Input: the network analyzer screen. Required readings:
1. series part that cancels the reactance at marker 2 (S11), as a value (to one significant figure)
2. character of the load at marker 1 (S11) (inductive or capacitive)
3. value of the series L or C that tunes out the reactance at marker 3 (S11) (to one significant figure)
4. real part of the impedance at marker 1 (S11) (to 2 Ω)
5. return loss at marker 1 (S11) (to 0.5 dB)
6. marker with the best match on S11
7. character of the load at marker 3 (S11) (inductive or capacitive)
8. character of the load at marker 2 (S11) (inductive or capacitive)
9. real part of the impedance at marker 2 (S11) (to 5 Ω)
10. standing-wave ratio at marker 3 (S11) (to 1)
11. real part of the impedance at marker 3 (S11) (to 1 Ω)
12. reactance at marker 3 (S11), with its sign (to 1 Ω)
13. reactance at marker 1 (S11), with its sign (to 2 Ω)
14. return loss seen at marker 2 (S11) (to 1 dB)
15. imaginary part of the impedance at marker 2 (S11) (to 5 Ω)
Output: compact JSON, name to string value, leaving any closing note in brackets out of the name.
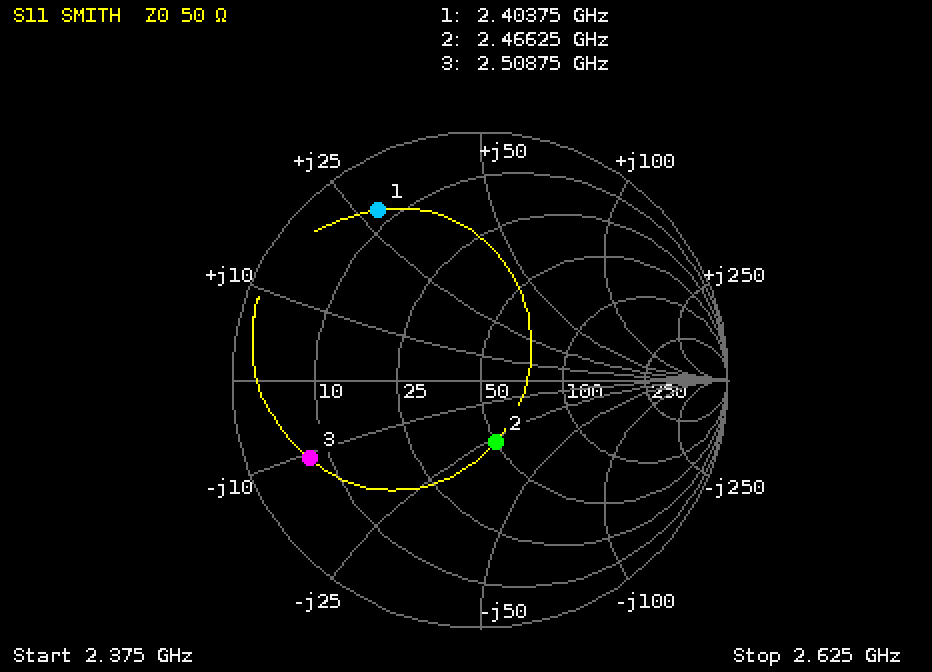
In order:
{"series part that cancels the reactance at marker 2 (S11), as a value": "2 nH", "character of the load at marker 1 (S11)": "inductive", "value of the series L or C that tunes out the reactance at marker 3 (S11)": "700 pH", "real part of the impedance at marker 1 (S11)": "8 Ω", "return loss at marker 1 (S11)": "2.0 dB", "marker with the best match on S11": "marker 2", "character of the load at marker 3 (S11)": "capacitive", "character of the load at marker 2 (S11)": "capacitive", "real part of the impedance at marker 2 (S11)": "50 Ω", "standing-wave ratio at marker 3 (S11)": "7", "real part of the impedance at marker 3 (S11)": "7 Ω", "reactance at marker 3 (S11), with its sign": "-11 Ω", "reactance at marker 1 (S11), with its sign": "+28 Ω", "return loss seen at marker 2 (S11)": "12 dB", "imaginary part of the impedance at marker 2 (S11)": "-25 Ω"}
